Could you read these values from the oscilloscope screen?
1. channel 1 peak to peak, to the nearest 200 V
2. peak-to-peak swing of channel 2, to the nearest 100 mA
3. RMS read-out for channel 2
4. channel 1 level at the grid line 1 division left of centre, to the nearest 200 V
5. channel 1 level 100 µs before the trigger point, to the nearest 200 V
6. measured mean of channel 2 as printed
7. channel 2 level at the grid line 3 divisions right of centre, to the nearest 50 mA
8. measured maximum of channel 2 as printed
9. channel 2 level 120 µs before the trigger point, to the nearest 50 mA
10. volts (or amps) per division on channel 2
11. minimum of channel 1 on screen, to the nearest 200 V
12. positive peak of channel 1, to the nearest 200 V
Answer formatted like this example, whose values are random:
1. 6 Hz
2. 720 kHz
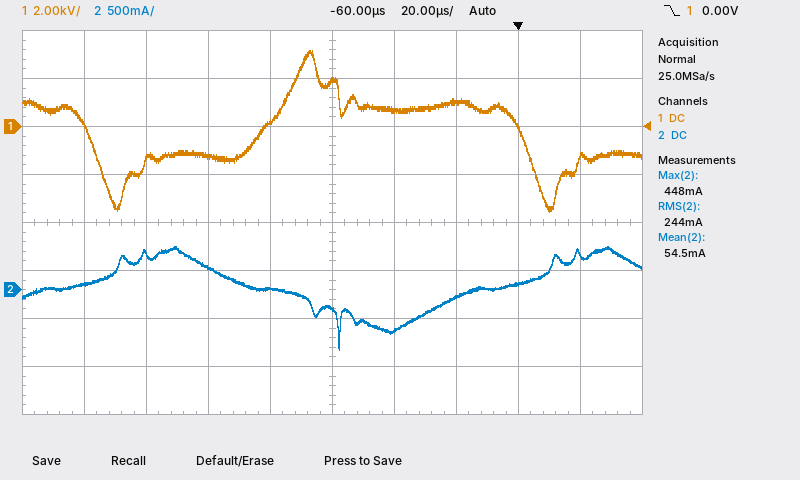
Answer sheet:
1. 6.8 kV
2. 1.10 A
3. 244 mA
4. 200 V
5. -1.2 kV
6. 54.5 mA
7. 50 mA
8. 448 mA
9. 350 mA
10. 500 mA
11. -3.6 kV
12. 3.2 kV
